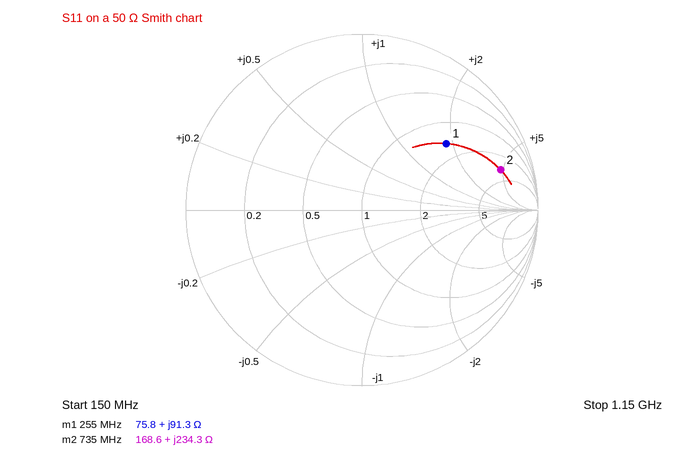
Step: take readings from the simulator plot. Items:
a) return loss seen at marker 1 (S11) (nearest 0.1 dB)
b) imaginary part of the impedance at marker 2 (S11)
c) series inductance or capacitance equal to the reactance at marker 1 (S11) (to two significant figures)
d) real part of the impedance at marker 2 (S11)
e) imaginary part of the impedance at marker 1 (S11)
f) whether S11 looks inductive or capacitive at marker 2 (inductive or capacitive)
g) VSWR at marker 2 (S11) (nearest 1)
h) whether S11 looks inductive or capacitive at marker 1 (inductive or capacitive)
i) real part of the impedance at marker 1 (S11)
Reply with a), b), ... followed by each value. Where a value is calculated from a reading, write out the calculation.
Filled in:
a) 4.3 dB
b) +234.3 Ω
c) L = 91.3 Ω/(2π × 255 MHz) ≈ 57 nH
d) 168.6 Ω
e) +91.3 Ω
f) inductive
g) 10
h) inductive
i) 75.8 Ω
